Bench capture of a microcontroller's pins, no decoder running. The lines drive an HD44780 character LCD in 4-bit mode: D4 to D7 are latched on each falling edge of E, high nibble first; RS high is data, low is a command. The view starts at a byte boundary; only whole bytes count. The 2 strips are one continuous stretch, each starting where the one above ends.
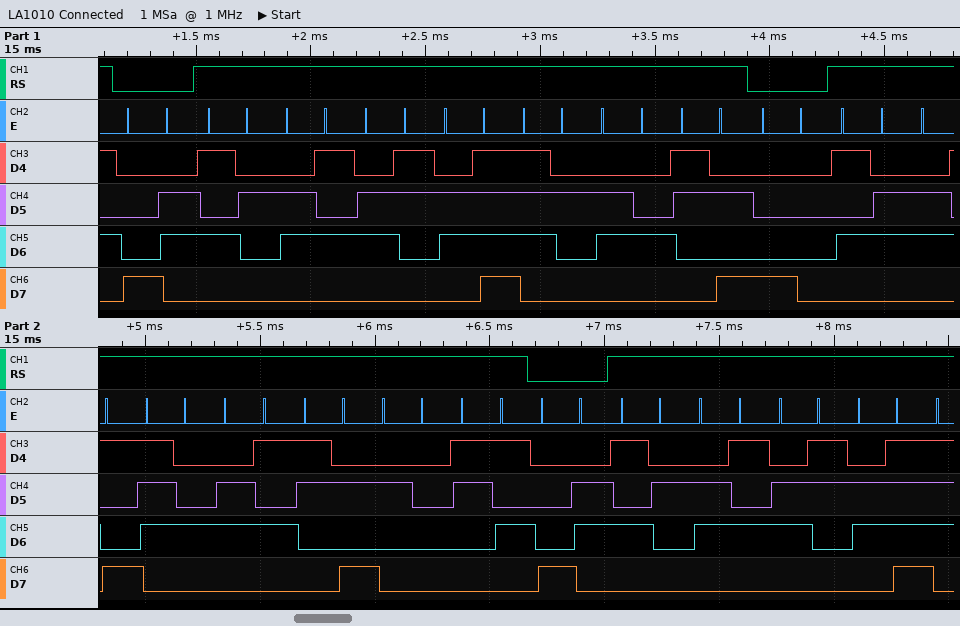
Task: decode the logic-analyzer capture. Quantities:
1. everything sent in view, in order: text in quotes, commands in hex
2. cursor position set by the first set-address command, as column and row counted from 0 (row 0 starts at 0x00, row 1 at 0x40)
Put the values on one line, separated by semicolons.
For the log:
0x86 "Record:" 0x80 "Vite: 5" 0x86 "Reco"; column 6, row 0
